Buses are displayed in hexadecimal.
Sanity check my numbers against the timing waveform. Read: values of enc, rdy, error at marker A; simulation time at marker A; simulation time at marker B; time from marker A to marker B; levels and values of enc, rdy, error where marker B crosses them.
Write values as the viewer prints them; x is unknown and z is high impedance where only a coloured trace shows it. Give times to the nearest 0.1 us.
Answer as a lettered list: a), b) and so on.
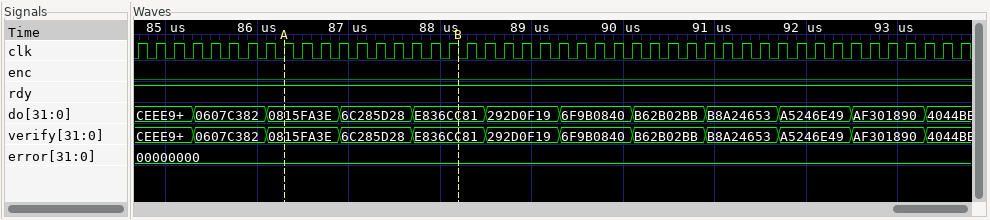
a) enc=0, rdy=1, error=00000000
b) 86.3 us
c) 88.2 us
d) 1.9 us
e) enc=0, rdy=1, error=00000000
